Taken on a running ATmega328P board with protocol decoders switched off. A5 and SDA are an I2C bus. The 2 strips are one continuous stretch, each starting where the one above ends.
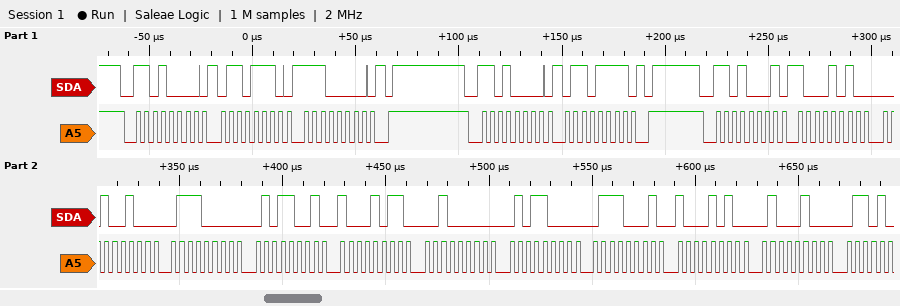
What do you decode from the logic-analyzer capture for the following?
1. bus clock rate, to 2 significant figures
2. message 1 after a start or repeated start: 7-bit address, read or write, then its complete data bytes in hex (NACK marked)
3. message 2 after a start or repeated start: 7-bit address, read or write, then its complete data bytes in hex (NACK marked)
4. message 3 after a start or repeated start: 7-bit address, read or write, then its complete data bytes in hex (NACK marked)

250 kHz
0x68 write: 6E E0
0x68 write: 6F
0x68 read: 8A 24 70 59 8B 20 58 71 8A 44
